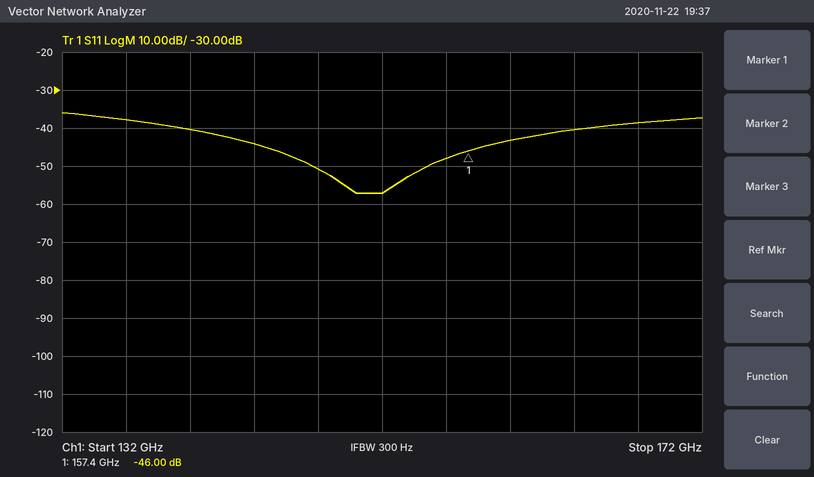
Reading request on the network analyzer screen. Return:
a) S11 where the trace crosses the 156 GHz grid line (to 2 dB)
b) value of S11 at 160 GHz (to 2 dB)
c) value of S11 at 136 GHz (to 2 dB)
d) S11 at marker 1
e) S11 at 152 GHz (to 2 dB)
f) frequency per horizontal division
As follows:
-48 dB
-44 dB
-38 dB
-46.00 dB
-58 dB
4 GHz
